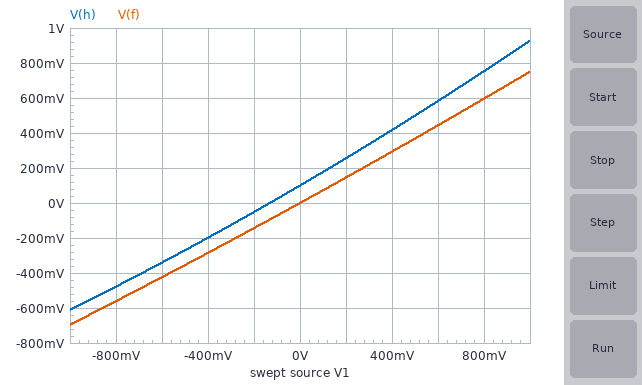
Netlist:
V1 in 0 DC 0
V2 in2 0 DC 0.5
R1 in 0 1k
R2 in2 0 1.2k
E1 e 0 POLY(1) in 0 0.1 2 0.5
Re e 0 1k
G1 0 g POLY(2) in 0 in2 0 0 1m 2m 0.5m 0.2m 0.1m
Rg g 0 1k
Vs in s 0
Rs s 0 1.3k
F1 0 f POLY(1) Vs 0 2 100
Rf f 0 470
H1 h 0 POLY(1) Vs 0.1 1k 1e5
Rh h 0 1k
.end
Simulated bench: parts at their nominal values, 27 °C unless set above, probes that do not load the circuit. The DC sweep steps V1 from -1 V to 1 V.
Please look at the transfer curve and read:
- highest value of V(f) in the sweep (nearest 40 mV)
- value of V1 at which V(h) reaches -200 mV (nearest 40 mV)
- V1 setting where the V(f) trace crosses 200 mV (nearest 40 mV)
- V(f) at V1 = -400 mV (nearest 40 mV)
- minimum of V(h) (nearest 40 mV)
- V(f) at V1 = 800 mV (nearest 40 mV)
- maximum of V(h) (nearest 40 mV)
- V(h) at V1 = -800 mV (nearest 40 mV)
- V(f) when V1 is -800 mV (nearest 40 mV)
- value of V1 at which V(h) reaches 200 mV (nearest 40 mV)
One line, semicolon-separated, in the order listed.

760 mV; -400 mV; 280 mV; -280 mV; -600 mV; 600 mV; 920 mV; -480 mV; -560 mV; 120 mV
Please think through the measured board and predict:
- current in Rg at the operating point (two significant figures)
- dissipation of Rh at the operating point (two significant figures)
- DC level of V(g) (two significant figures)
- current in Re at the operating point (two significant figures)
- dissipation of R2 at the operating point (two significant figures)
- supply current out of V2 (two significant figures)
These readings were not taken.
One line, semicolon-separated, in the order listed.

1.0 mA; 10 µW; 1.0 V; 100 µA; 210 µW; 420 µA
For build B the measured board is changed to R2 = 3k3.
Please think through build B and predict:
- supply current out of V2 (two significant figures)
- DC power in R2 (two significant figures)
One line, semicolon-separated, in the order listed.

150 µA; 76 µW
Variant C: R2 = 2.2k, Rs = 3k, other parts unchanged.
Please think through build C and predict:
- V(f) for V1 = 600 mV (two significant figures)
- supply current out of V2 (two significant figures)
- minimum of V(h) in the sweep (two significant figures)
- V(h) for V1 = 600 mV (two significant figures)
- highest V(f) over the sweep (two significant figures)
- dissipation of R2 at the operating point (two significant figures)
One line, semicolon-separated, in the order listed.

190 mV; 230 µA; -220 mV; 300 mV; 320 mV; 110 µW
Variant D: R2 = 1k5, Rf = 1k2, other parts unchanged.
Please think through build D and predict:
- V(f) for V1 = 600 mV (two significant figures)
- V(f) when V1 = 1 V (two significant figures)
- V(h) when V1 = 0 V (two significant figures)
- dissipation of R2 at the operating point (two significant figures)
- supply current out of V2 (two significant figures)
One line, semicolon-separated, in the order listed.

1.1 V; 1.9 V; 100 mV; 170 µW; 330 µA
